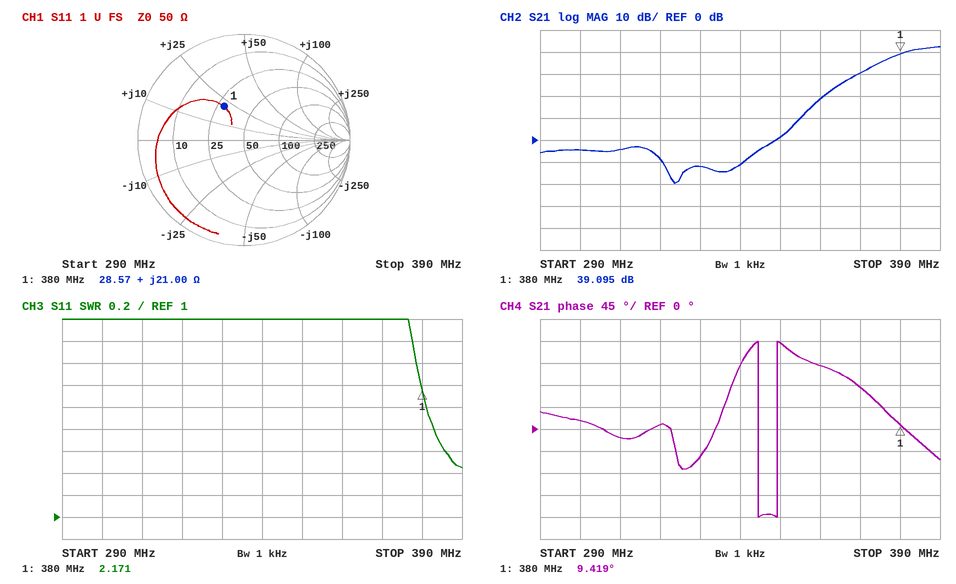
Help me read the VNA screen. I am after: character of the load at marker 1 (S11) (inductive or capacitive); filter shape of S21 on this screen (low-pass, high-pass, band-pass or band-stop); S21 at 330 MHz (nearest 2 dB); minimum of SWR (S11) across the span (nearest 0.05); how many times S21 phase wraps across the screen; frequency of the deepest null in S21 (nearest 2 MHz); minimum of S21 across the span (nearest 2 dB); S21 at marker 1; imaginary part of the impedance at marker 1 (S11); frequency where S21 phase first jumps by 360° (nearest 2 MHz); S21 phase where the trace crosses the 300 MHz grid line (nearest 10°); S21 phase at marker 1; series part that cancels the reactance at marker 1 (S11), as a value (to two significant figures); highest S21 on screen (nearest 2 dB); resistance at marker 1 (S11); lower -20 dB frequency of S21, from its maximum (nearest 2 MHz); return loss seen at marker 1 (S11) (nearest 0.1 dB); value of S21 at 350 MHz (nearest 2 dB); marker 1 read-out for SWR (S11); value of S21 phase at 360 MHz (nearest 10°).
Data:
inductive
high-pass
-12 dB
1.45
2
324 MHz
-20 dB
39.095 dB
+21.00 Ω
344 MHz
20°
9.419°
20 pF
42 dB
28.57 Ω
362 MHz
8.7 dB
2 dB
2.171
130°
